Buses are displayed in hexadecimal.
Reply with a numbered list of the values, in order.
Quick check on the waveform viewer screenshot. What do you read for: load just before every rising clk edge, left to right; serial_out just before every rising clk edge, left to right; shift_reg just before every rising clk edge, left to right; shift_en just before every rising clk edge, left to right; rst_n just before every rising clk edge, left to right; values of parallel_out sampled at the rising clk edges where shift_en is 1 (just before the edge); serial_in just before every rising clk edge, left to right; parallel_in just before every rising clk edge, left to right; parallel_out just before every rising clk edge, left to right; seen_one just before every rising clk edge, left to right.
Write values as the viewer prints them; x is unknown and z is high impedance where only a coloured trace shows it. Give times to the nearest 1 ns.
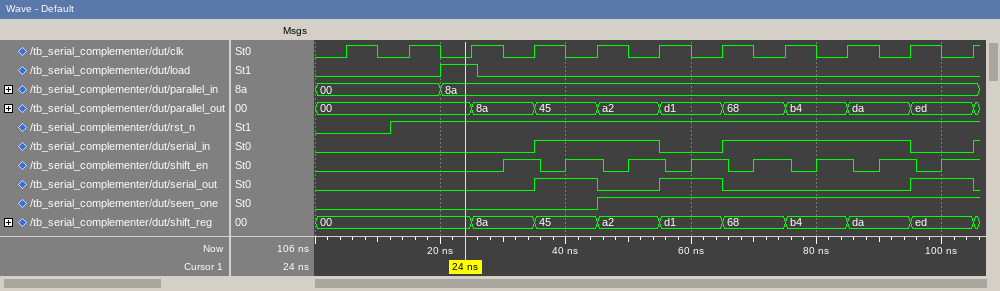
1. 0 0 1 0 0 0 0 0 0 0 0
2. 0 0 0 0 1 0 1 0 0 0 1
3. 00, 00, 00, 8a, 45, a2, d1, 68, b4, da, ed
4. 0 0 0 1 1 1 1 1 1 1 1
5. 0 1 1 1 1 1 1 1 1 1 1
6. 8a, 45, a2, d1, 68, b4, da, ed
7. 0 0 0 0 1 1 0 1 1 1 0
8. 00, 00, 8a, 8a, 8a, 8a, 8a, 8a, 8a, 8a, 8a
9. 00, 00, 00, 8a, 45, a2, d1, 68, b4, da, ed
10. 0 0 0 0 0 1 1 1 1 1 1
